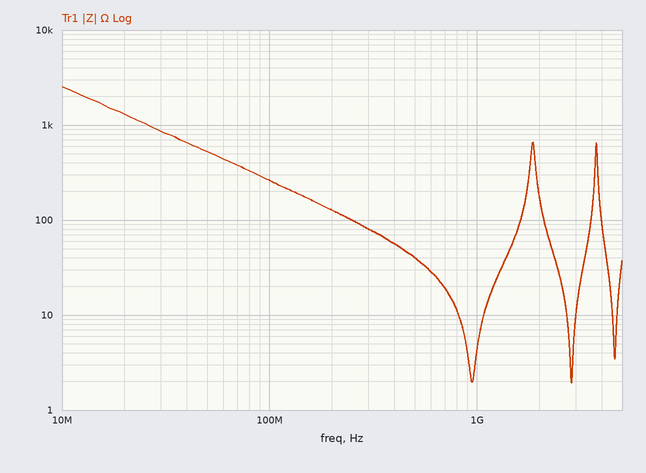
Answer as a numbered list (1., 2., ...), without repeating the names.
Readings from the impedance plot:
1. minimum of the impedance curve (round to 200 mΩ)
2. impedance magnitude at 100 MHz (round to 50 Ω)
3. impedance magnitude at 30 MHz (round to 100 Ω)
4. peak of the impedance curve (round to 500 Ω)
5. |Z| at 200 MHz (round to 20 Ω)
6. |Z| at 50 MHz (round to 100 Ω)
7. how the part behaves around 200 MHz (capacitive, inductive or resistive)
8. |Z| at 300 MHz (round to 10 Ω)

1. 2.0 Ω
2. 250 Ω
3. 900 Ω
4. 2.5 kΩ
5. 120 Ω
6. 500 Ω
7. capacitive
8. 80 Ω
